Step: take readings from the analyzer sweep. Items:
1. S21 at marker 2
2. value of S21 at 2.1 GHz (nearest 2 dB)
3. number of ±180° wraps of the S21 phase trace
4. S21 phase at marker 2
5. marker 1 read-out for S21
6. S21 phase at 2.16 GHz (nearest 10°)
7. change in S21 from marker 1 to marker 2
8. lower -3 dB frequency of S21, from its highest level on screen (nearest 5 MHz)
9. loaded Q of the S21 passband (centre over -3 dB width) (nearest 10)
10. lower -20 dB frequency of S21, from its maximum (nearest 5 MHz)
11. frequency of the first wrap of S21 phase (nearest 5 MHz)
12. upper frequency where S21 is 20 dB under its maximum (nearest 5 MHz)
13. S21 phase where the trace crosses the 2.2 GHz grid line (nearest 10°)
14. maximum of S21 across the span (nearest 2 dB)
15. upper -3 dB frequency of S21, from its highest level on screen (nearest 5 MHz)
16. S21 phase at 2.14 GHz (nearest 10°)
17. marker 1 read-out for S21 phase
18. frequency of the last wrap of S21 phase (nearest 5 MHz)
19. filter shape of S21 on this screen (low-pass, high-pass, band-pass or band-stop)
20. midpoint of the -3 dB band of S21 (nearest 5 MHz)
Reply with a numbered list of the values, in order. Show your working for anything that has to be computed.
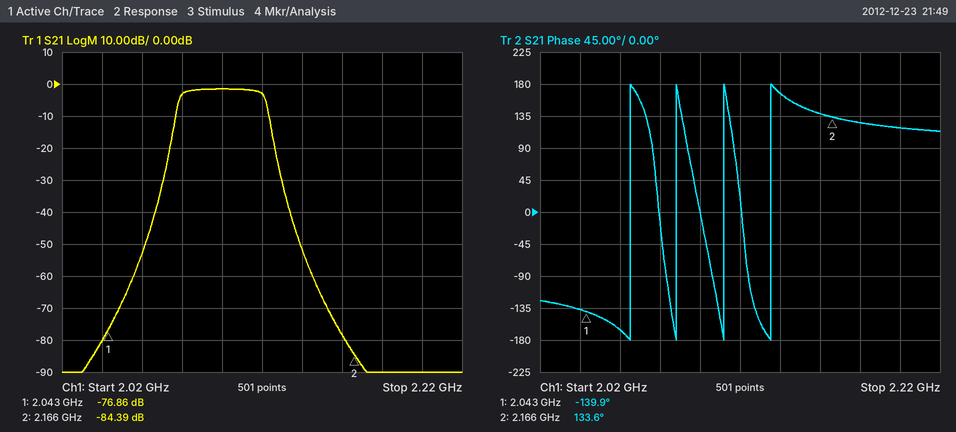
1. -84.39 dB
2. -2 dB
3. 4
4. 133.6°
5. -76.86 dB
6. 140°
7. -84.39 − (-76.86) = -7.53 dB
8. 2.080 GHz
9. 2.1 GHz / 40 MHz ≈ 52.5, so 50 to the nearest 10
10. 2.075 GHz
11. 2.065 GHz
12. 2.125 GHz
13. 120°
14. -2 dB
15. 2.120 GHz
16. 170°
17. -139.9°
18. 2.135 GHz
19. band-pass
20. 2.100 GHz
